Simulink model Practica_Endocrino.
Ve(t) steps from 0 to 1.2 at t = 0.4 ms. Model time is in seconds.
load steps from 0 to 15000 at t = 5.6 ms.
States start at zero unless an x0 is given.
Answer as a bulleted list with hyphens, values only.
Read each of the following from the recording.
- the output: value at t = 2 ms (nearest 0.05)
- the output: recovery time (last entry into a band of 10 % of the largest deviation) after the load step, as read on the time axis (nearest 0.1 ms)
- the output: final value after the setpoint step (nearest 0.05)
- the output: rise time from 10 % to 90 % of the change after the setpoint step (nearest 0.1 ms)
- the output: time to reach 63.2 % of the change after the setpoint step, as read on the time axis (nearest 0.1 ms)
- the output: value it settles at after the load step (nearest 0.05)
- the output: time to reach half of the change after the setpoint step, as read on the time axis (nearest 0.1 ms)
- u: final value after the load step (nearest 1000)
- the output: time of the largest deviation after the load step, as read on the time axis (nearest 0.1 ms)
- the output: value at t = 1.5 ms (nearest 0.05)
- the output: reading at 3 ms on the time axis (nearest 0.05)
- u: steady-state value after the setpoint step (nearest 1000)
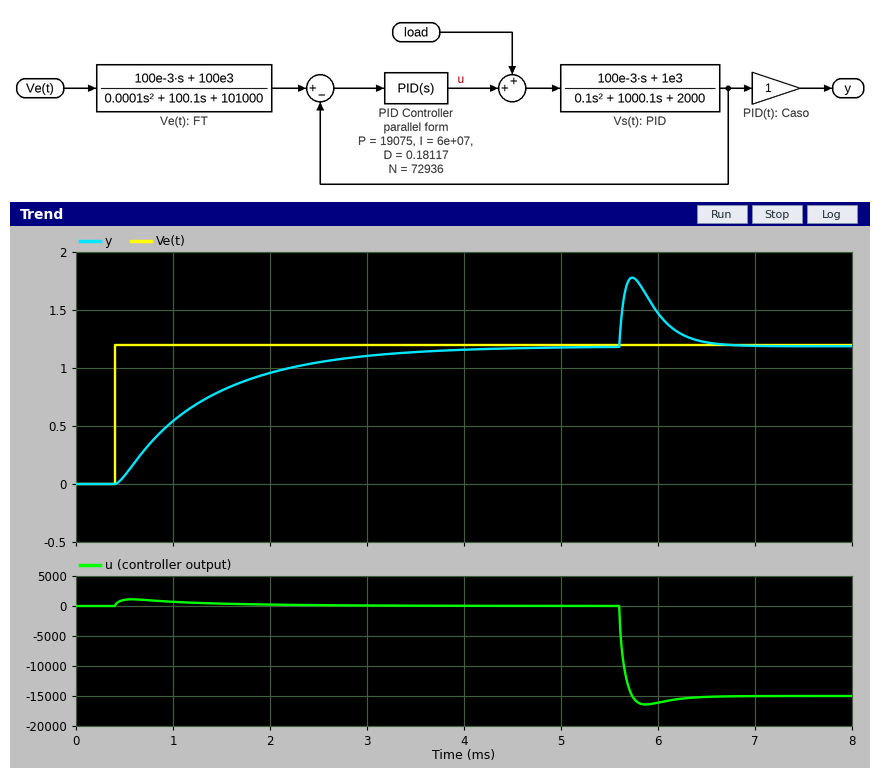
- 0.95
- 6.4 ms
- 1.20
- 2.1 ms
- 1.4 ms
- 1.20
- 1.1 ms
- -15000
- 5.7 ms
- 0.80
- 1.10
- 0
